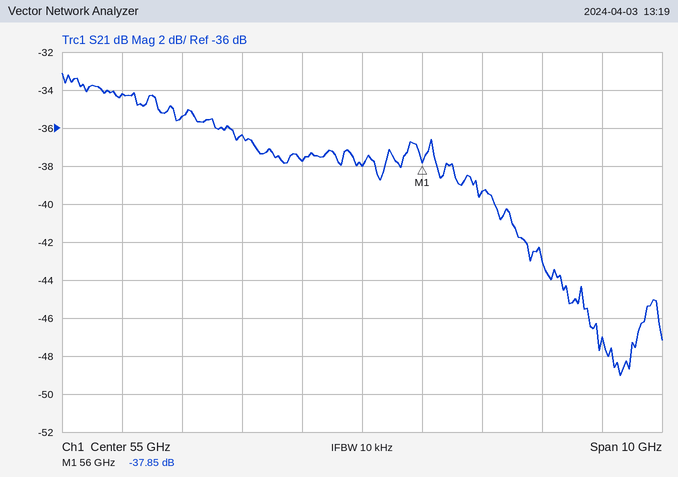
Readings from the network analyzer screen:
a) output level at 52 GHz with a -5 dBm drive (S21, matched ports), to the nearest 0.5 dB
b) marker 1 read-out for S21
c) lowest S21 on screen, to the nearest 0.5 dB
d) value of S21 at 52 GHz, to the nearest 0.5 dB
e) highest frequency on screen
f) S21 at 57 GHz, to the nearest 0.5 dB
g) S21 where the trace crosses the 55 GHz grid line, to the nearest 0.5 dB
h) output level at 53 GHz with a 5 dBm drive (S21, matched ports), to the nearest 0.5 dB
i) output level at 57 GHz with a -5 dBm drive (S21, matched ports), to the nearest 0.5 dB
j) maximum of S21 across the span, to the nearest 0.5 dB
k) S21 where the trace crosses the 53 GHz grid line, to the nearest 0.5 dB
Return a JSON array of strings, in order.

["-40.5 dBm", "-37.85 dB", "-49.0 dB", "-35.5 dB", "60 GHz", "-39.5 dB", "-38.0 dB", "-31.5 dBm", "-44.5 dBm", "-33.0 dB", "-36.5 dB"]
